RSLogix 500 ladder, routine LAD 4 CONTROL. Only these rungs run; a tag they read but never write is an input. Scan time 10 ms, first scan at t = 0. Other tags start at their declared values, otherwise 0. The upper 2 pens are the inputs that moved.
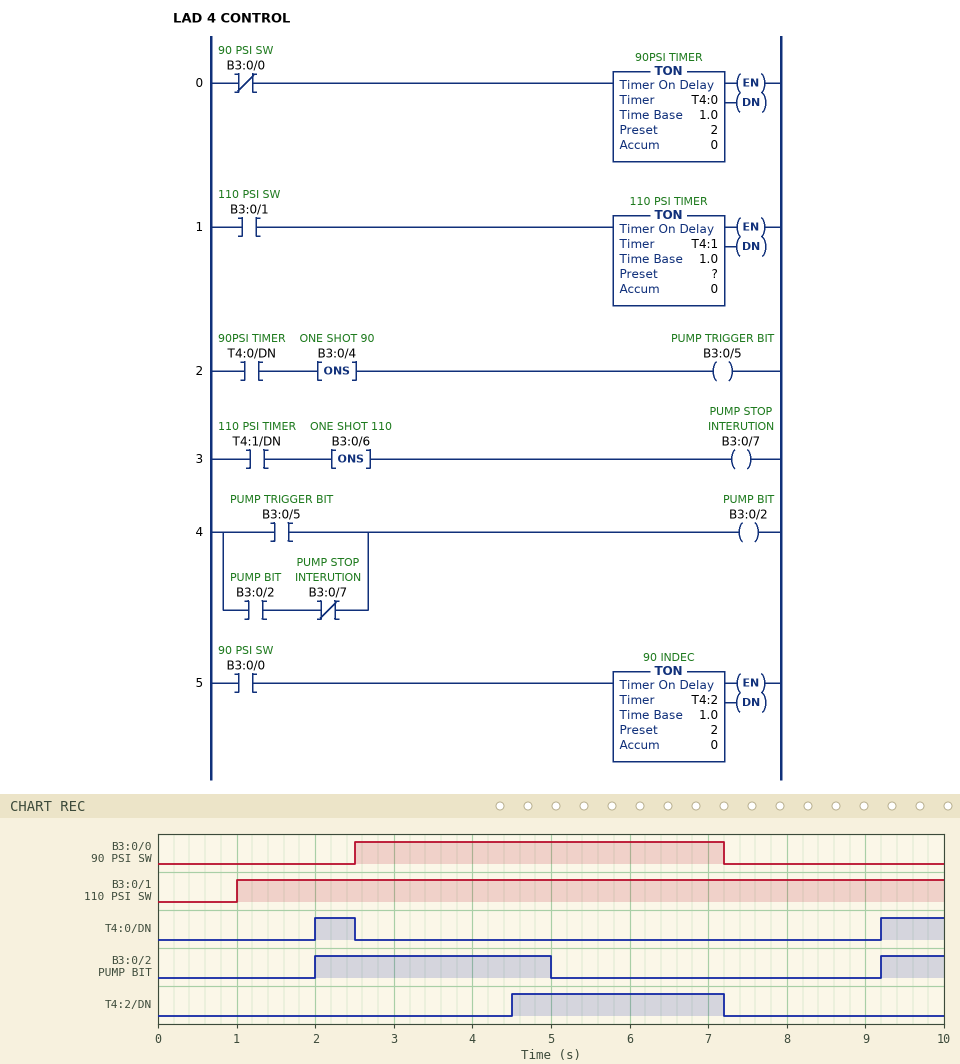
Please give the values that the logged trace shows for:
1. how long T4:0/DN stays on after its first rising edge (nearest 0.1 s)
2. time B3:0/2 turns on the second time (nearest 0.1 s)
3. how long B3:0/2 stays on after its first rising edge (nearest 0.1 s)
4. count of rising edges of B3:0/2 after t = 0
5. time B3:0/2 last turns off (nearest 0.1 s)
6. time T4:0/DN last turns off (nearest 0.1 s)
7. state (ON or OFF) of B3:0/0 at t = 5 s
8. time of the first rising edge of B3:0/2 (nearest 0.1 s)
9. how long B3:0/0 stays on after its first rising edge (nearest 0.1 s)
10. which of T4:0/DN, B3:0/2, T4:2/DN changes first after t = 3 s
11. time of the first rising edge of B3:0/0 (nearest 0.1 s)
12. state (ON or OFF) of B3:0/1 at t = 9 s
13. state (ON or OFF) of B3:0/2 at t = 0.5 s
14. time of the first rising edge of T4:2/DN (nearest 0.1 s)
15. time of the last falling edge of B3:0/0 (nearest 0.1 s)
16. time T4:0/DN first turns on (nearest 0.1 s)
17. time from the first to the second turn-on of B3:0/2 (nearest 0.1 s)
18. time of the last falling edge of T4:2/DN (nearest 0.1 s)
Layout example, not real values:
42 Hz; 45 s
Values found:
0.5 s; 9.2 s; 3.0 s; 2; 5.0 s; 2.5 s; ON; 2.0 s; 4.7 s; T4:2/DN; 2.5 s; ON; OFF; 4.5 s; 7.2 s; 2.0 s; 7.2 s; 7.2 s
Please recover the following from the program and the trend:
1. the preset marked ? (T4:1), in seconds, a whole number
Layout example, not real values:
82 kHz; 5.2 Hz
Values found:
4 s
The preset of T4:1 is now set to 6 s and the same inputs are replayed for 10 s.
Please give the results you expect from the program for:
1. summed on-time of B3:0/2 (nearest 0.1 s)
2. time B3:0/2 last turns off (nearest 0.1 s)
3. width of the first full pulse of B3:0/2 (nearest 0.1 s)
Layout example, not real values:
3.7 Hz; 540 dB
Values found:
5.8 s; 7.0 s; 5.0 s
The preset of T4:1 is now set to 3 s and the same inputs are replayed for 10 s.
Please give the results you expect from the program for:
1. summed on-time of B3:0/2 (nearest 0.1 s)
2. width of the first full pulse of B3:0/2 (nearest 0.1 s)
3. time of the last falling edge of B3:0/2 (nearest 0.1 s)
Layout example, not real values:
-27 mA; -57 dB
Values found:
2.8 s; 2.0 s; 4.0 s
